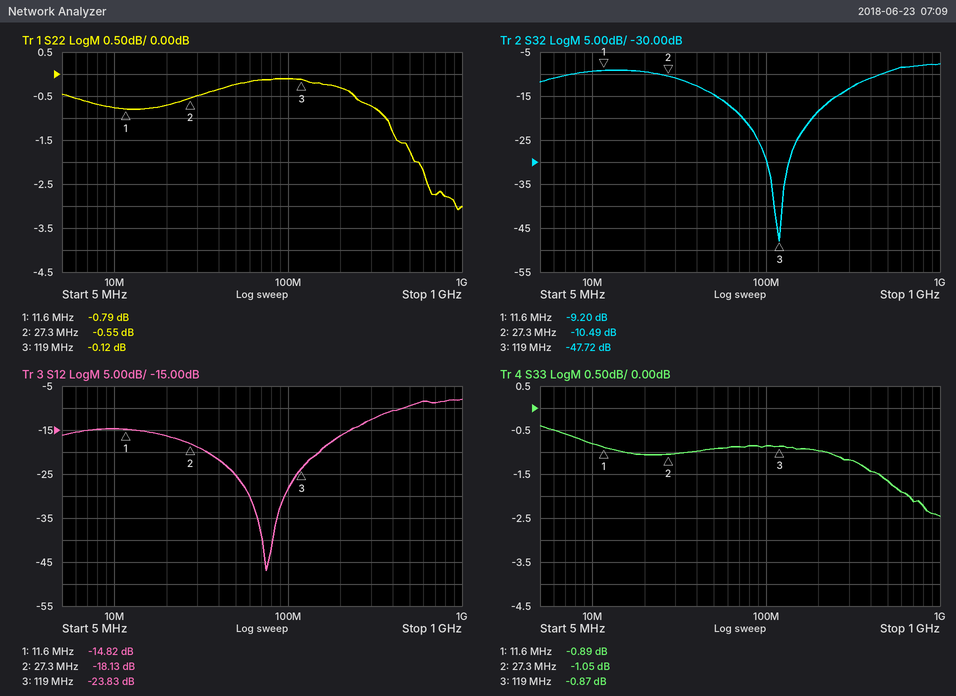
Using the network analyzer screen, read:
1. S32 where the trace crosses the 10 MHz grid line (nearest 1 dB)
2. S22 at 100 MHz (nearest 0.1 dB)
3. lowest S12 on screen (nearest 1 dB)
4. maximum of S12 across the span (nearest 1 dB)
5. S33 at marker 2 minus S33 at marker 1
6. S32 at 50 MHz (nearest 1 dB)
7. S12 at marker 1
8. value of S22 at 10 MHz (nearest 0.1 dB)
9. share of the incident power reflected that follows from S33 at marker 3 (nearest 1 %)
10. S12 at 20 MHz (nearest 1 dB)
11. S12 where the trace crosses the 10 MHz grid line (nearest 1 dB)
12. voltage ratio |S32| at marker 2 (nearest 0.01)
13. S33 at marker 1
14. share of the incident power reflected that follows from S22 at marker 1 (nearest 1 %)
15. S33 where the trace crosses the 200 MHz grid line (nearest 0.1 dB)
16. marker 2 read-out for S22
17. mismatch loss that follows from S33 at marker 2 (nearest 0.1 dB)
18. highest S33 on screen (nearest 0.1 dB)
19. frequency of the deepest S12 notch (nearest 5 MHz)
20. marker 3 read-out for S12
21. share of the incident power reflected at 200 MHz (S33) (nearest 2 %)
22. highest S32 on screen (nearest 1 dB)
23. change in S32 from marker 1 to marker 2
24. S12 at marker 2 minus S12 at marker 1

-9 dB
-0.1 dB
-47 dB
-8 dB
-0.16 dB
-15 dB
-14.82 dB
-0.8 dB
82 %
-16 dB
-15 dB
0.30
-0.89 dB
83 %
-1.0 dB
-0.55 dB
6.7 dB
-0.4 dB
75 MHz
-23.83 dB
80 %
-8 dB
-1.29 dB
-3.31 dB
